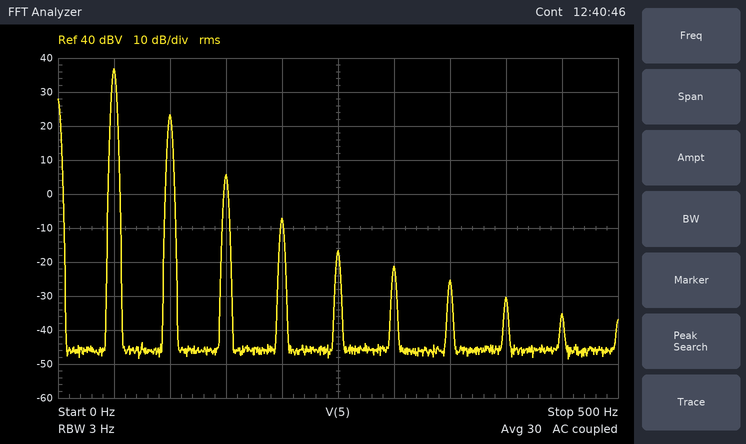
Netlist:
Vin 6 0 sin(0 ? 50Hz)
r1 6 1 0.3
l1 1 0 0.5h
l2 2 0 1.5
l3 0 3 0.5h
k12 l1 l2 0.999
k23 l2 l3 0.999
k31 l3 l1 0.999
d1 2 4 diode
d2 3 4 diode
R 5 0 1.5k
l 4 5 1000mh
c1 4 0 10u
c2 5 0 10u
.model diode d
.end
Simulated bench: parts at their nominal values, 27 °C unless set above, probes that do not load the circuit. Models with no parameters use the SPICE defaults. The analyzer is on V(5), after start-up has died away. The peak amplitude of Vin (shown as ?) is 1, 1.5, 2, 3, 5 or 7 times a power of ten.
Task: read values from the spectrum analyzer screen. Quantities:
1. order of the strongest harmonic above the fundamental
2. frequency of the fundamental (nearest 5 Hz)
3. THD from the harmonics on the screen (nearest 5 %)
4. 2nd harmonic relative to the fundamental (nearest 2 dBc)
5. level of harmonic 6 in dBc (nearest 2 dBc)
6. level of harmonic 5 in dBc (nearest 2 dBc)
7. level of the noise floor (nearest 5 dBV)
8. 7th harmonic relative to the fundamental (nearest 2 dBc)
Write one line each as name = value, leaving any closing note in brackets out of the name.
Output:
order of the strongest harmonic above the fundamental = 2
frequency of the fundamental = 50 Hz
THD from the harmonics on the screen = 20 %
2nd harmonic relative to the fundamental = -14 dBc
level of harmonic 6 in dBc = -58 dBc
level of harmonic 5 in dBc = -54 dBc
level of the noise floor = -45 dBV
7th harmonic relative to the fundamental = -62 dBc
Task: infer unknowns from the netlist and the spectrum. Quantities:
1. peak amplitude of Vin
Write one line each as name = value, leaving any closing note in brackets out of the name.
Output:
peak amplitude of Vin = 200 V
